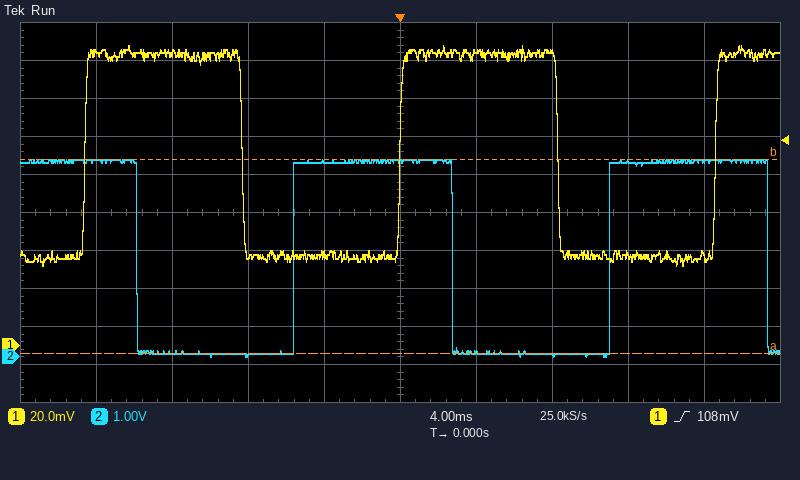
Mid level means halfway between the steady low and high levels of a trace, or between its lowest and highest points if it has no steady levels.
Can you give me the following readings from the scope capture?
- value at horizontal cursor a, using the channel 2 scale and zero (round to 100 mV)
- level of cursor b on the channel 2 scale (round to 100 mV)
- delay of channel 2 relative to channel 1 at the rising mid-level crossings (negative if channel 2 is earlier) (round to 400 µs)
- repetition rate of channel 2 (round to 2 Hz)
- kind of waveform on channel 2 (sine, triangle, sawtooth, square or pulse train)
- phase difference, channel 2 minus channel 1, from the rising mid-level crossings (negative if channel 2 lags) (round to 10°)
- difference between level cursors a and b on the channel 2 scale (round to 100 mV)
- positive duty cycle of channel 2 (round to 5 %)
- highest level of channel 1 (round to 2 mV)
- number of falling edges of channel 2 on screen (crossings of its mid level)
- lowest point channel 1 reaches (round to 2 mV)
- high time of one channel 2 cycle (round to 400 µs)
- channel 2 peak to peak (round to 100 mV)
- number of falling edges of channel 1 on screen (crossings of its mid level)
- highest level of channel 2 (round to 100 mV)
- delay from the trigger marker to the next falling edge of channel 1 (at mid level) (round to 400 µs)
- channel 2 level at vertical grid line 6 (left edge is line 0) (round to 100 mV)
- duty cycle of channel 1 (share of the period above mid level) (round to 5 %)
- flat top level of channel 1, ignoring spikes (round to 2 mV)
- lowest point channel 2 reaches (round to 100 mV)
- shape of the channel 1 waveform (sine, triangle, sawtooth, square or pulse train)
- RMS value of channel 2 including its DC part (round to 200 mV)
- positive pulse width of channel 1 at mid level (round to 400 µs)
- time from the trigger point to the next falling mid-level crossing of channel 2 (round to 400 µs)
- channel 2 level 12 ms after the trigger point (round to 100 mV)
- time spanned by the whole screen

100 mV
5.2 V
-5.6 ms
60 Hz
square
+120°
5.1 V
50 %
158 mV
3
42 mV
8.4 ms
5.2 V
2
5.2 V
8.4 ms
100 mV
50 %
154 mV
0.0 V
square
3.6 V
8.4 ms
2.8 ms
5.2 V
40 ms
